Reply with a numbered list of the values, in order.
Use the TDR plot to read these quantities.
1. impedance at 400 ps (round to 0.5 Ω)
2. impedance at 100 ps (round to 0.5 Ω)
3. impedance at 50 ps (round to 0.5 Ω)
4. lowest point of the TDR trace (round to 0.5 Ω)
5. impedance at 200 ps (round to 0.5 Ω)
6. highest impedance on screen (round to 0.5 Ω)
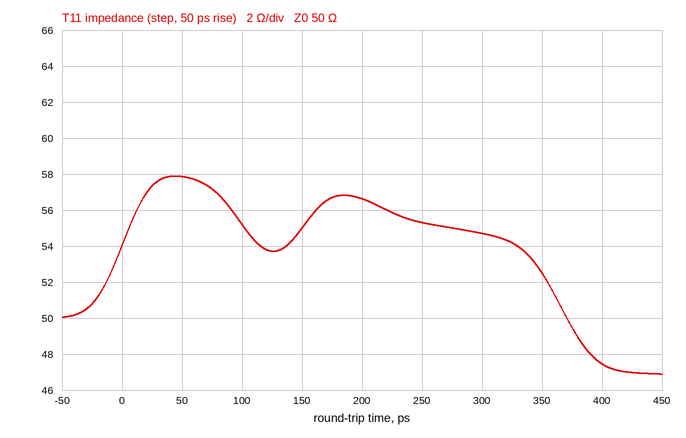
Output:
1. 47.5 Ω
2. 55.0 Ω
3. 58.0 Ω
4. 47.0 Ω
5. 56.5 Ω
6. 58.0 Ω
